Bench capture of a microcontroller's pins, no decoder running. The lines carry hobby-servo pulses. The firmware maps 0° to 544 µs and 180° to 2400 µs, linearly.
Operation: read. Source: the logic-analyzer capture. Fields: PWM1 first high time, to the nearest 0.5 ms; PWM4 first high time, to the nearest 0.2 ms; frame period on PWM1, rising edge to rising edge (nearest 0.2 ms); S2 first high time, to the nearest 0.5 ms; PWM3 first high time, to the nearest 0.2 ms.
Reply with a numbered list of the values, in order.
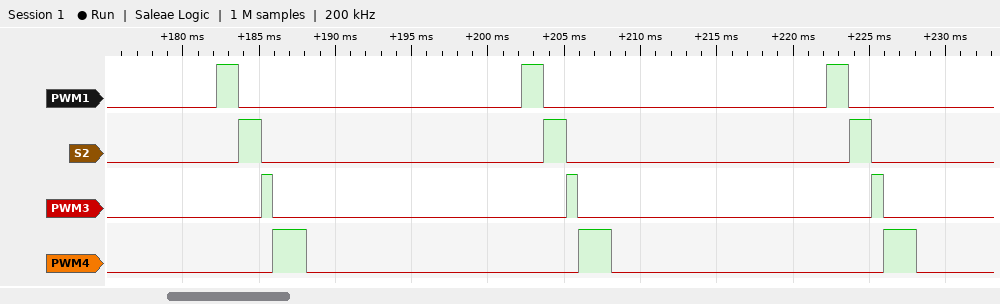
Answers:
1. 1.5 ms
2. 2.2 ms
3. 20.0 ms
4. 1.5 ms
5. 0.8 ms
